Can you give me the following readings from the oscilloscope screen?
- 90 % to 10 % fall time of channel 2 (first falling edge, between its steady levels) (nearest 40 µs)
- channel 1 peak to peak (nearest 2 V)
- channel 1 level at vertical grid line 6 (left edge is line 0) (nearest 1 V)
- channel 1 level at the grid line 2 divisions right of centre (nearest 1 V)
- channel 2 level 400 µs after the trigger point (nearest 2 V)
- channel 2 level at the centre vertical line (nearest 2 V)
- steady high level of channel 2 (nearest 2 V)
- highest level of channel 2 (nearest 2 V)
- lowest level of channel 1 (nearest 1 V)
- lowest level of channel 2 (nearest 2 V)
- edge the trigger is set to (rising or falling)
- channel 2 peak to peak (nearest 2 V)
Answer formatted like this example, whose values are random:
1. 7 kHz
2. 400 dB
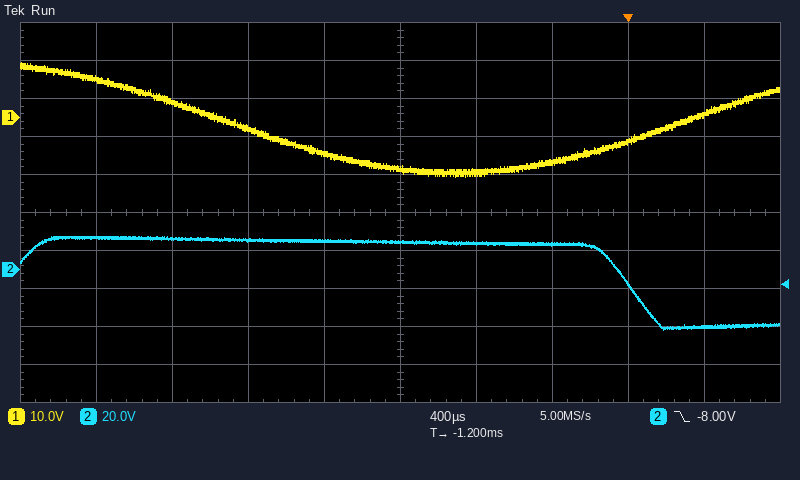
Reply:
1. 280 µs
2. 30 V
3. -14 V
4. -12 V
5. -30 V
6. 14 V
7. 14 V
8. 18 V
9. -16 V
10. -32 V
11. falling
12. 50 V
